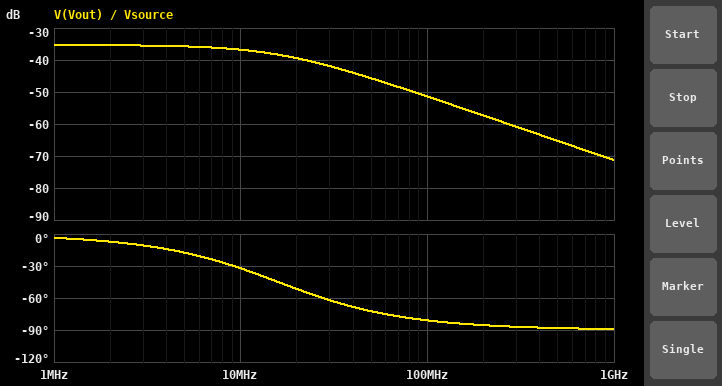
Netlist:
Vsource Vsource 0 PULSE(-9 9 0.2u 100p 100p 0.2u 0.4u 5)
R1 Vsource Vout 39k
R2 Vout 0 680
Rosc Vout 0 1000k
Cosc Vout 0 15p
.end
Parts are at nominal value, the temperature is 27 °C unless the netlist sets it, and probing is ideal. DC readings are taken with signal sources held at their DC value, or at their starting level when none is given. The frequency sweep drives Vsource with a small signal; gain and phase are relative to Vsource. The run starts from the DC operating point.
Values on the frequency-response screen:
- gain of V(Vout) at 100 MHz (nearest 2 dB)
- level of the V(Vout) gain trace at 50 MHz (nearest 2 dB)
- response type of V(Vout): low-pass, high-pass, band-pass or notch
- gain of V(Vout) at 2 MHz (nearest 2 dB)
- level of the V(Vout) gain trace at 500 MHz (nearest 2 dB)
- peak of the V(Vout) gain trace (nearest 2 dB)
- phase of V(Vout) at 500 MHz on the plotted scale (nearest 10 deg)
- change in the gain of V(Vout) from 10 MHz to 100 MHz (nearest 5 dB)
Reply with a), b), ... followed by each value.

a) -52 dB
b) -46 dB
c) low-pass
d) -36 dB
e) -66 dB
f) -36 dB
g) -90 deg
h) -15 dB
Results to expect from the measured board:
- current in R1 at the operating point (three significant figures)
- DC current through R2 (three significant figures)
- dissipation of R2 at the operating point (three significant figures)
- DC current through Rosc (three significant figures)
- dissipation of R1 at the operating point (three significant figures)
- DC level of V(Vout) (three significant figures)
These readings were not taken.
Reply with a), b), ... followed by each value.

a) 227 µA
b) 227 µA
c) 34.9 µW
d) 154 nA
e) 2.01 mW
f) -154 mV
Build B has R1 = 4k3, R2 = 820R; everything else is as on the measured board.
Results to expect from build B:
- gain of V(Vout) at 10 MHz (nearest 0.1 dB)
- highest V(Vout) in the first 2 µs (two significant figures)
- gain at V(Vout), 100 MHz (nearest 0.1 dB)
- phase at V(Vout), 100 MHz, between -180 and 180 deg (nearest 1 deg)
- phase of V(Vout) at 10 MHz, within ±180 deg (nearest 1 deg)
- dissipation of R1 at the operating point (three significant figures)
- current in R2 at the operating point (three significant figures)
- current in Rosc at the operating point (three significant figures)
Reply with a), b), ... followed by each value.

a) -17.4 dB
b) 1.4 V
c) -32.3 dB
d) -81 deg
e) -33 deg
f) 13.3 mW
g) 1.76 mA
h) 1.44 µA
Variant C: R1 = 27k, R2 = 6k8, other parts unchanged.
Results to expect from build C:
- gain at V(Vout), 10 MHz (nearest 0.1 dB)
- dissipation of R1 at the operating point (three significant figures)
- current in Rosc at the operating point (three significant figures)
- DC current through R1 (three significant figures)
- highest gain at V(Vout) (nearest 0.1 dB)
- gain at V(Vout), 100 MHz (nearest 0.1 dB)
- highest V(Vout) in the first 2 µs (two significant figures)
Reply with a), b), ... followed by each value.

a) -28.3 dB
b) 1.92 mW
c) 1.80 µA
d) 267 µA
e) -14.0 dB
f) -48.1 dB
g) 1.5 V
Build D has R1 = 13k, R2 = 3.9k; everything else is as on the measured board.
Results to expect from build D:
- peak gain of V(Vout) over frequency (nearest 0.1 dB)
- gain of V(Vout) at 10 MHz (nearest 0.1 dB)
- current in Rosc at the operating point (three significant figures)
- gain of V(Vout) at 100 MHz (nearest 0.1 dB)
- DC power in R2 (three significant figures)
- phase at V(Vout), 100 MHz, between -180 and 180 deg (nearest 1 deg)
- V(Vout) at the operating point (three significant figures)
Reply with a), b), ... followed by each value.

a) -12.8 dB
b) -22.3 dB
c) 2.07 µA
d) -41.8 dB
e) 1.10 mW
f) -88 deg
g) -2.07 V
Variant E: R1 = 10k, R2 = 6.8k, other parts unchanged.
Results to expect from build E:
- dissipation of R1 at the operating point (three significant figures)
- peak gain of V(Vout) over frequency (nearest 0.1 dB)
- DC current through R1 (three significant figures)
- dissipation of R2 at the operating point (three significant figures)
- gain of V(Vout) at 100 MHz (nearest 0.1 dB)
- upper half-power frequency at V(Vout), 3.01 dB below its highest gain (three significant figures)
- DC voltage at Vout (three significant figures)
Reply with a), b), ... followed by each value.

a) 2.89 mW
b) -7.9 dB
c) 537 µA
d) 1.94 mW
e) -39.5 dB
f) 2.63 MHz
g) -3.63 V
